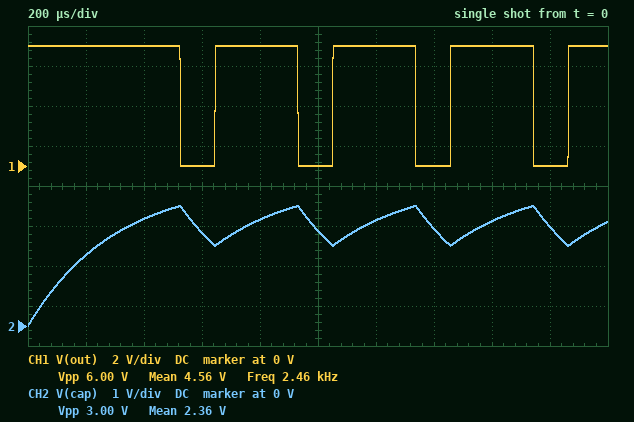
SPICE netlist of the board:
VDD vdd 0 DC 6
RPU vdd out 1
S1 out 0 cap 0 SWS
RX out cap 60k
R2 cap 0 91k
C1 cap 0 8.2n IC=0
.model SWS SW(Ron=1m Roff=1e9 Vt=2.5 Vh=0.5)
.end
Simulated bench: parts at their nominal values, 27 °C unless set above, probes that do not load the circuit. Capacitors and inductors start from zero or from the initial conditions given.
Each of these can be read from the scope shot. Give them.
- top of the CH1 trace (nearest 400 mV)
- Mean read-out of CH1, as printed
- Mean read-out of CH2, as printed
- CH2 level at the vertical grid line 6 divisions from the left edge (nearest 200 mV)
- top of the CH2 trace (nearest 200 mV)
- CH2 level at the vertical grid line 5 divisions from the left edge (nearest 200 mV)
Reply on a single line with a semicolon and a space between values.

6.0 V; 4.56 V; 2.36 V; 2.6 V; 3.0 V; 2.4 V
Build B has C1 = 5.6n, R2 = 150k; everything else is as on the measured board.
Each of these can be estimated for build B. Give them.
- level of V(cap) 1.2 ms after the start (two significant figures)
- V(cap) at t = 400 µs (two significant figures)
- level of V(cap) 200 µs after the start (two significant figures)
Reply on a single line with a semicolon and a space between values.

2.8 V; 2.1 V; 2.4 V
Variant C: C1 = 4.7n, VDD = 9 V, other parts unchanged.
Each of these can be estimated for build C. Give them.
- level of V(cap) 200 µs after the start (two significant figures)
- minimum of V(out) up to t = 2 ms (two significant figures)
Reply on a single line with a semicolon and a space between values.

2.1 V; 9.0 mV
